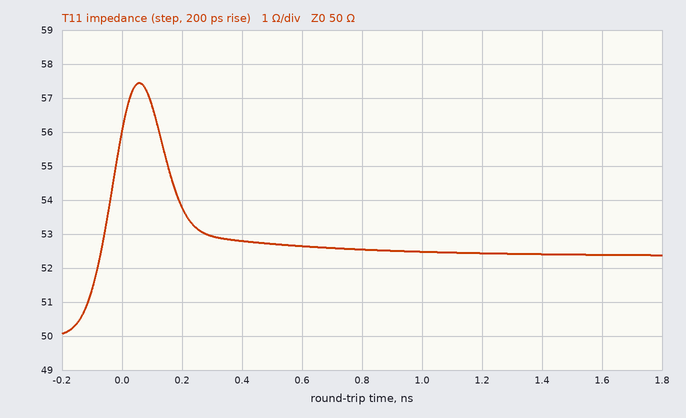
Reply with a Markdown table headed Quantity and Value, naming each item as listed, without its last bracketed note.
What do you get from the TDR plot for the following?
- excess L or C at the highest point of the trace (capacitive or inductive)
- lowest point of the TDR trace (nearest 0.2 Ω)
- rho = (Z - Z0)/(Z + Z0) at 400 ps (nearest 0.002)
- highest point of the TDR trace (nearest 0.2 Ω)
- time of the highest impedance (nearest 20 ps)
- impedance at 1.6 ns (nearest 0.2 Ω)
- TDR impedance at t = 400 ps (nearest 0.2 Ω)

| Quantity | Value |
|---|---|
| excess L or C at the highest point of the trace | inductive |
| lowest point of the TDR trace | 50.0 Ω |
| rho = (Z - Z0)/(Z + Z0) at 400 ps | +0.028 |
| highest point of the TDR trace | 57.4 Ω |
| time of the highest impedance | 60 ps |
| impedance at 1.6 ns | 52.4 Ω |
| TDR impedance at t = 400 ps | 52.8 Ω |
